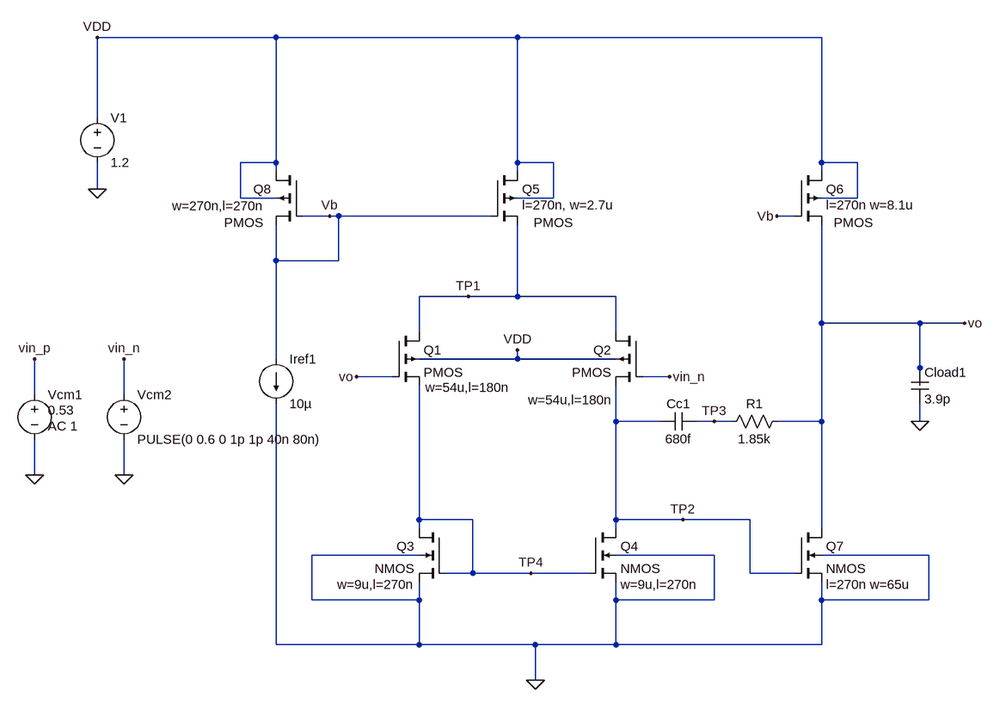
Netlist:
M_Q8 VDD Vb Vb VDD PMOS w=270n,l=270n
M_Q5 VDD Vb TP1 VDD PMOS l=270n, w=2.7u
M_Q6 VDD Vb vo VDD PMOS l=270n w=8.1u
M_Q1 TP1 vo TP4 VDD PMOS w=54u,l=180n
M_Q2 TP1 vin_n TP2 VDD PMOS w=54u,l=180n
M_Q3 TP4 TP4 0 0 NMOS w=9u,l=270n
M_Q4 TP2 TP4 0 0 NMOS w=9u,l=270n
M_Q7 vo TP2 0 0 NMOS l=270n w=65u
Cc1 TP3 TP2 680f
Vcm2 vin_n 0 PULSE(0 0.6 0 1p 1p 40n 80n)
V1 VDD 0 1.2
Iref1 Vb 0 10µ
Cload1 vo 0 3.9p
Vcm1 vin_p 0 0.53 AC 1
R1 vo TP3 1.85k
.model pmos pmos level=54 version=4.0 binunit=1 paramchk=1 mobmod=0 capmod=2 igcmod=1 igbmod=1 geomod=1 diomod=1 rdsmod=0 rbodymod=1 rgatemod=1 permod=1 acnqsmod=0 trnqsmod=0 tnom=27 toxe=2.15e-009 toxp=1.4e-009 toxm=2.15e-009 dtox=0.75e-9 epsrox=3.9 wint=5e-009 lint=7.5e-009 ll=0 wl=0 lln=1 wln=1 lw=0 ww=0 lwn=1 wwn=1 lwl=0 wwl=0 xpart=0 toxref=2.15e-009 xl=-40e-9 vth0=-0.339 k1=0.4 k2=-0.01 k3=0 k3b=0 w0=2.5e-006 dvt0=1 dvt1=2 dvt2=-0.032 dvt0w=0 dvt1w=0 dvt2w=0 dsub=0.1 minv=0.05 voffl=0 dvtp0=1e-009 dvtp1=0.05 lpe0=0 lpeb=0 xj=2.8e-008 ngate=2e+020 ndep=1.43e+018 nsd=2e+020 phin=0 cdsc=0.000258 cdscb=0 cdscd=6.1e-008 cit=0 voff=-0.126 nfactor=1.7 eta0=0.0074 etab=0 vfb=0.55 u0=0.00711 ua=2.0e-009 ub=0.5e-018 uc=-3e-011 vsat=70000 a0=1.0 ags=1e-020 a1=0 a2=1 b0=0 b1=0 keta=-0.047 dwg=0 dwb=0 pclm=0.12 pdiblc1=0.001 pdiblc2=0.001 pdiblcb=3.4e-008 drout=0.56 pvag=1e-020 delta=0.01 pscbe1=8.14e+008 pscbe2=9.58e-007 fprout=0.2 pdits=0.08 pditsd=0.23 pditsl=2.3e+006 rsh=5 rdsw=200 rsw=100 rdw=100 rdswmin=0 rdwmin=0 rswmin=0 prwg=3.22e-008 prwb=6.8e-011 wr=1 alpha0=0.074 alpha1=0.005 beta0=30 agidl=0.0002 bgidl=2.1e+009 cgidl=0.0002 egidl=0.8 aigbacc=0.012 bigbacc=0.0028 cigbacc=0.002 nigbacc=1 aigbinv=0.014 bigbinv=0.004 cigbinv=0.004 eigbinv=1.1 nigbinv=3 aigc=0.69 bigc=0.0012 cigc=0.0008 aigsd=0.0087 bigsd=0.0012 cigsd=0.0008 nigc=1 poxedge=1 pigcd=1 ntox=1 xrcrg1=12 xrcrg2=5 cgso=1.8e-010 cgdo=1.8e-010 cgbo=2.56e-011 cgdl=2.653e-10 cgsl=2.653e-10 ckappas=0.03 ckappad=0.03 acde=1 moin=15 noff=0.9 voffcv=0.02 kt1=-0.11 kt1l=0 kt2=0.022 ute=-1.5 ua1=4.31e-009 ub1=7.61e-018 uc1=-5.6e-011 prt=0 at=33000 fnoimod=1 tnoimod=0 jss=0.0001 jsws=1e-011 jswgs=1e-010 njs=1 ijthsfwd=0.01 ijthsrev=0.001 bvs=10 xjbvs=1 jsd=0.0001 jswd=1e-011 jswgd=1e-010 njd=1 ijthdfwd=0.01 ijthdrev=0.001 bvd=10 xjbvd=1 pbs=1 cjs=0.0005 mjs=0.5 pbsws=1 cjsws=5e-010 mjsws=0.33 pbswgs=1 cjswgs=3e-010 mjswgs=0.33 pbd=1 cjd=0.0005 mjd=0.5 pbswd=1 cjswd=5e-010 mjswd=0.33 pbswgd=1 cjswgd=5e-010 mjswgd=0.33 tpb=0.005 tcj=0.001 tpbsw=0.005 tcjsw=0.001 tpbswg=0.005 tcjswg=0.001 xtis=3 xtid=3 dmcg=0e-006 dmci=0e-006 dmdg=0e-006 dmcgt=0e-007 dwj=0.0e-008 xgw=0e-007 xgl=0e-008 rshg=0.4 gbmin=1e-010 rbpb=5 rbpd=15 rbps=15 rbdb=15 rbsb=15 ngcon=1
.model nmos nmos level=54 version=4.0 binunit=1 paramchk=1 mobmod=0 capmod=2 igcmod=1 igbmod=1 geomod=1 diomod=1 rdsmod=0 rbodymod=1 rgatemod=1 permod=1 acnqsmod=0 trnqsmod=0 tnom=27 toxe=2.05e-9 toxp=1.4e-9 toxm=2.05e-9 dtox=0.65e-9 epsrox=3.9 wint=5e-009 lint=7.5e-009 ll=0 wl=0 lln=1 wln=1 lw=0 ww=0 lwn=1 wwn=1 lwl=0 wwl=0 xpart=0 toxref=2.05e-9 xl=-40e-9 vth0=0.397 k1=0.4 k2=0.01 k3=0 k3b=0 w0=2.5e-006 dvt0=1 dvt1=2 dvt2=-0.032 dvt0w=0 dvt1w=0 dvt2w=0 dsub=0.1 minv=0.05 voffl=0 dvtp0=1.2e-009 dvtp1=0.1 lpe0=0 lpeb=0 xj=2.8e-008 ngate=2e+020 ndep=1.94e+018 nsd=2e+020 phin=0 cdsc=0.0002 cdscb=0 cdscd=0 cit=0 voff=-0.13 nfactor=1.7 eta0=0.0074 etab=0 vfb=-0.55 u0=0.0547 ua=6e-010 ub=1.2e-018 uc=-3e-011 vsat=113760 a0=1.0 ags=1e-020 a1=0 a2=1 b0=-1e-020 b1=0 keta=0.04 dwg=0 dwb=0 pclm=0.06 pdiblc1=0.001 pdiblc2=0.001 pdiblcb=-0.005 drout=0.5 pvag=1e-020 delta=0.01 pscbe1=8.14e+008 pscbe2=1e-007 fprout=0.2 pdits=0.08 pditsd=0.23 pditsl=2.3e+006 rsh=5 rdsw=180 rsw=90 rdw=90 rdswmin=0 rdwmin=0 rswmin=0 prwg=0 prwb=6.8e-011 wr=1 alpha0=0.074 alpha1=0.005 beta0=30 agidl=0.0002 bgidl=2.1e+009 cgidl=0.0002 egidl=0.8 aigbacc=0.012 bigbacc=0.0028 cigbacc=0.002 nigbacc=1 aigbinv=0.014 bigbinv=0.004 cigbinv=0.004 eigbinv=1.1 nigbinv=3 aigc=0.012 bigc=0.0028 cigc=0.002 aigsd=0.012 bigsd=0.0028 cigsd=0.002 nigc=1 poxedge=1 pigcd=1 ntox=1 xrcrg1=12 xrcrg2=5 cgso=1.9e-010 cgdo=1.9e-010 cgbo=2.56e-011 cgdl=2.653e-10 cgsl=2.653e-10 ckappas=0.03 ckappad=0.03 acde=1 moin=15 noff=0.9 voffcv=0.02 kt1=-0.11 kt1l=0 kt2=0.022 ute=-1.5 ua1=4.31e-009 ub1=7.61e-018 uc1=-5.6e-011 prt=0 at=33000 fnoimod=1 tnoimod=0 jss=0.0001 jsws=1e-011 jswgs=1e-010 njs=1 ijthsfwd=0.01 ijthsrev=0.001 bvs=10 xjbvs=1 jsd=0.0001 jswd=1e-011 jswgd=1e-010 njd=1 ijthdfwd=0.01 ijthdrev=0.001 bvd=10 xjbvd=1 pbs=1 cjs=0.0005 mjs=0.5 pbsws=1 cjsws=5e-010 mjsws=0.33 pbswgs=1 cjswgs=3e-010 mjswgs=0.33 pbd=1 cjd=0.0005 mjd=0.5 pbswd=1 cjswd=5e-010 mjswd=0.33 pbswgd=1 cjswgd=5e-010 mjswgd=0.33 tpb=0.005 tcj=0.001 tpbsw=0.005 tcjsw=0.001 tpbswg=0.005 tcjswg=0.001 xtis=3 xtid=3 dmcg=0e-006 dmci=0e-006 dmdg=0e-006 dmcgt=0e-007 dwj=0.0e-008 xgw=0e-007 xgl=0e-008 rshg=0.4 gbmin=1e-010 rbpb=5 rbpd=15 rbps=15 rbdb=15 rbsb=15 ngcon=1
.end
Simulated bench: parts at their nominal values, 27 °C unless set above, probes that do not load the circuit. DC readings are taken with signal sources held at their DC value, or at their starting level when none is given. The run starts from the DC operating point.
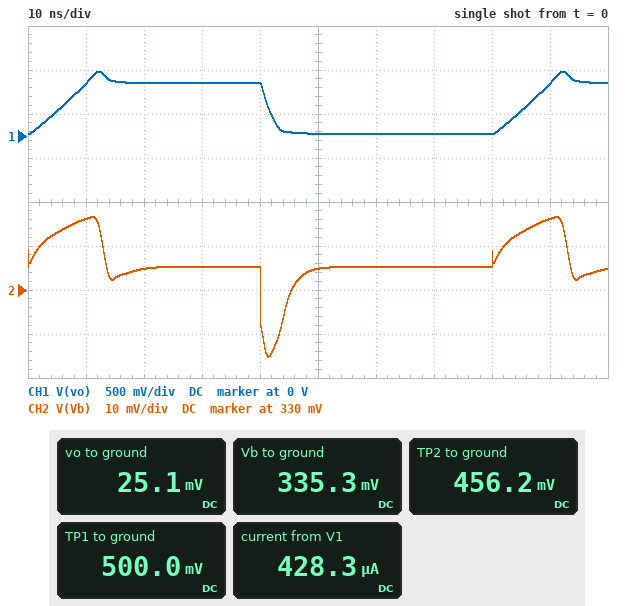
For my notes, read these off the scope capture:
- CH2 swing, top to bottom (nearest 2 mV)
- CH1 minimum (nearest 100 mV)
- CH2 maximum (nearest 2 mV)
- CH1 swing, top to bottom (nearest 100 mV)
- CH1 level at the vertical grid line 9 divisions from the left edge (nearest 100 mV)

32 mV
0 V
346 mV
700 mV
600 mV
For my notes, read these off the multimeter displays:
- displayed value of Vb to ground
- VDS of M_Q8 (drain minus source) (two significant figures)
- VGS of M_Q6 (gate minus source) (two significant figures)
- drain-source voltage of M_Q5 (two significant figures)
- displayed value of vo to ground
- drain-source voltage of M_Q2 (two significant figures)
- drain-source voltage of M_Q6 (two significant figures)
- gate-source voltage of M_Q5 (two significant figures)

335.3 mV
860 mV
310 mV
700 mV
25.1 mV
44 mV
1.2 V
-160 mV
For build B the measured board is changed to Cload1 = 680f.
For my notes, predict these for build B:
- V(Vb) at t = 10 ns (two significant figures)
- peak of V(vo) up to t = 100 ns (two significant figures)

340 mV
600 mV
